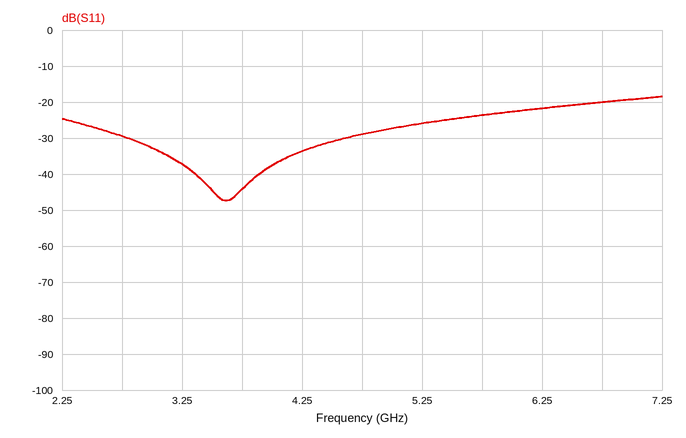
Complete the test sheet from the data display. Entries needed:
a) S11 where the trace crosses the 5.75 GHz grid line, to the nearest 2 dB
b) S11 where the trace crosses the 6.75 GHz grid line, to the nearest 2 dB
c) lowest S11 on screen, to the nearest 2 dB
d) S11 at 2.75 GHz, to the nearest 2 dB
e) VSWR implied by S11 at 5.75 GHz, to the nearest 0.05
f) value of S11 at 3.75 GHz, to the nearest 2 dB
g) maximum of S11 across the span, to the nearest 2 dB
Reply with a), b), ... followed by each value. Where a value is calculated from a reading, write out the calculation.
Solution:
a) -24 dB
b) -20 dB
c) -48 dB
d) -30 dB
e) |Γ| = 10^(-24/20) = 0.0631; VSWR = (1 + 0.0631)/(1 − 0.0631) ≈ 1.13, so 1.15 to the nearest 0.05
f) -44 dB
g) -18 dB
